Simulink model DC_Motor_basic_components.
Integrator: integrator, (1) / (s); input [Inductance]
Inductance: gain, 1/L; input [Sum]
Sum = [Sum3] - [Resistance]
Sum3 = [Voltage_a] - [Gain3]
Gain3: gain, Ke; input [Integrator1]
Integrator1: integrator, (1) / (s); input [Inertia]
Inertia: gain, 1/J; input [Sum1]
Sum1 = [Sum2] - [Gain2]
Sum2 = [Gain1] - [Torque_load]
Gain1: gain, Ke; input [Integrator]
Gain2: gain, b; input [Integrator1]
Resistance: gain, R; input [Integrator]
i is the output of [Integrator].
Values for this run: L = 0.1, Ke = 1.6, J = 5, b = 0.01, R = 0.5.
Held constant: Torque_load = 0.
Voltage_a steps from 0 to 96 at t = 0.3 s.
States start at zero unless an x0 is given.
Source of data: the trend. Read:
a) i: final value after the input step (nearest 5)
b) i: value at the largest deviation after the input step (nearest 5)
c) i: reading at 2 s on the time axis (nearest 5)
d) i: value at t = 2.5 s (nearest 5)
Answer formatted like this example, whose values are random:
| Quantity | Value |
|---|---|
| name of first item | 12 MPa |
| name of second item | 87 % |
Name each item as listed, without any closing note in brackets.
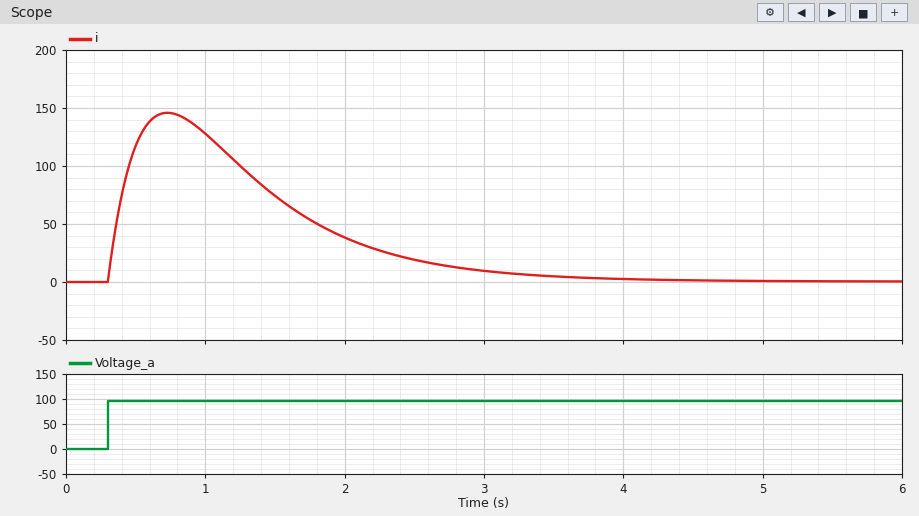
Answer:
| Quantity | Value |
|---|---|
| i: final value after the input step | 0 |
| i: value at the largest deviation after the input step | 145 |
| i: reading at 2 s on the time axis | 40 |
| i: value at t = 2.5 s | 20 |
